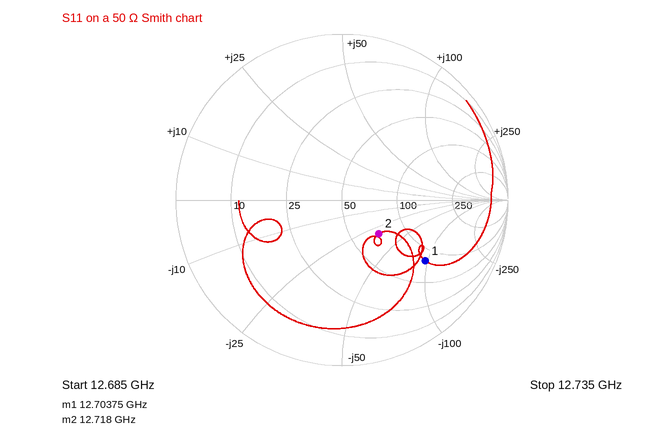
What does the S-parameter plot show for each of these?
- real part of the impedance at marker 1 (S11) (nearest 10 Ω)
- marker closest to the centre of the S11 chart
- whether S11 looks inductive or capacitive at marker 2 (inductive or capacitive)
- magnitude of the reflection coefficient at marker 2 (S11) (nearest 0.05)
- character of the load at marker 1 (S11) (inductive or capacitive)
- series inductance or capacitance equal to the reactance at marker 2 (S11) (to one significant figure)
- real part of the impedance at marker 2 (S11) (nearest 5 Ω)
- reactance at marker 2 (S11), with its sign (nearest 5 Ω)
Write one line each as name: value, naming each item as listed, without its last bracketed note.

real part of the impedance at marker 1 (S11): 80 Ω
marker closest to the centre of the S11 chart: marker 2
whether S11 looks inductive or capacitive at marker 2: capacitive
magnitude of the reflection coefficient at marker 2 (S11): 0.30
character of the load at marker 1 (S11): capacitive
series inductance or capacitance equal to the reactance at marker 2 (S11): 400 fF
real part of the impedance at marker 2 (S11): 70 Ω
reactance at marker 2 (S11), with its sign: -30 Ω
